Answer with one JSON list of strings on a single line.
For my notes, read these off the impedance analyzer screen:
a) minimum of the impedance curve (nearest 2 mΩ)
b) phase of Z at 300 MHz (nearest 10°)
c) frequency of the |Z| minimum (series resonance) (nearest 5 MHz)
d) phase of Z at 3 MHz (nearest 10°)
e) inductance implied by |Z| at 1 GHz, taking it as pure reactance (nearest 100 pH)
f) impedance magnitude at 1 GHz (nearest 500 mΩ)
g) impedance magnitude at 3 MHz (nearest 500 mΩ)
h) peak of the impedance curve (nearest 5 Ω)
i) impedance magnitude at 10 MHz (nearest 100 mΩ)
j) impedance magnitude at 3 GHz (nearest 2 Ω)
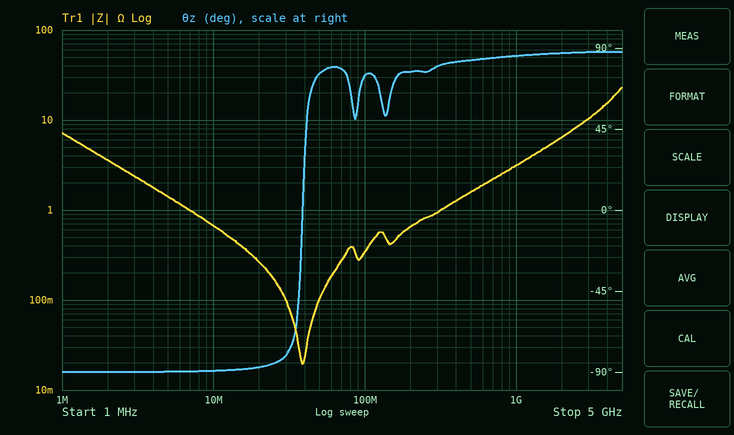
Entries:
["20 mΩ", "80°", "40 MHz", "-90°", "500 pH", "3.0 Ω", "2.5 Ω", "25 Ω", "700 mΩ", "10 Ω"]
